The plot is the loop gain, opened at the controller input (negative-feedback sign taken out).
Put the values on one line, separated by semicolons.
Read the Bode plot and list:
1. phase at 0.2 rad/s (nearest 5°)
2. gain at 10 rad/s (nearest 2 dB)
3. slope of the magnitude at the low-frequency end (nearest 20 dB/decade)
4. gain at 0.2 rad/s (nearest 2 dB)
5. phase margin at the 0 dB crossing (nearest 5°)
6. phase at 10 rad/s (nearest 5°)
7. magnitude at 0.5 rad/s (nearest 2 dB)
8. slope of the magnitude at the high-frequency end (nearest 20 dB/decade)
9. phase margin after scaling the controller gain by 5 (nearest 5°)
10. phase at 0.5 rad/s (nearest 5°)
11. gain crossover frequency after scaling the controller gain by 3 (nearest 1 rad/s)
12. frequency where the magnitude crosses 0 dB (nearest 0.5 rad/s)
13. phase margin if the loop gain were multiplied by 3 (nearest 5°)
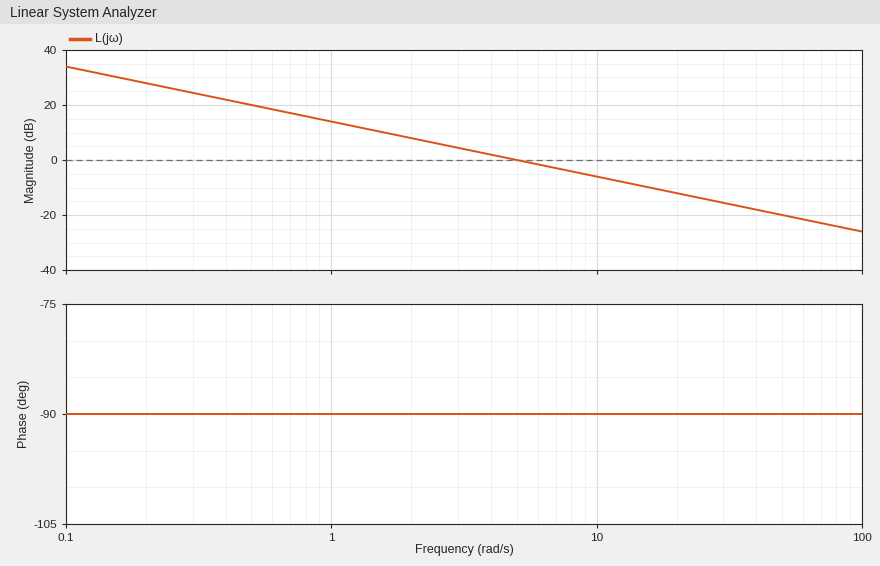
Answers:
-90°; -6 dB; -20 dB/decade; 28 dB; 90°; -90°; 20 dB; -20 dB/decade; 90°; -90°; 15 rad/s; 5.0 rad/s; 90°
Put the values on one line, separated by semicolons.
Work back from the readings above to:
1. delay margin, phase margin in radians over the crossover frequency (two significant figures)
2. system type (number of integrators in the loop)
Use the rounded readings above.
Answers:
0.31 s; 1
